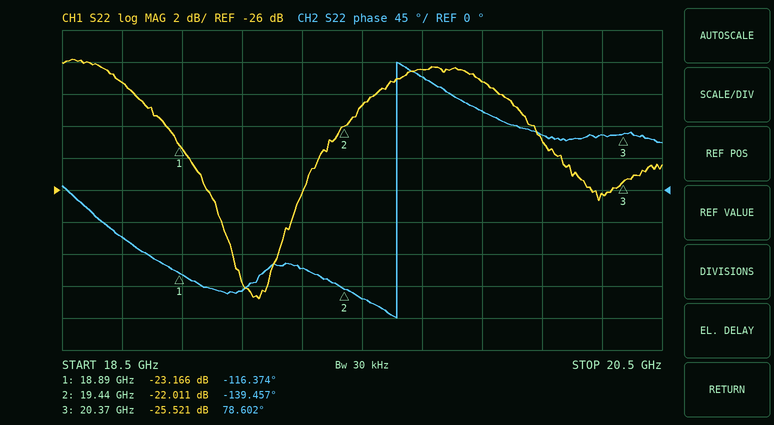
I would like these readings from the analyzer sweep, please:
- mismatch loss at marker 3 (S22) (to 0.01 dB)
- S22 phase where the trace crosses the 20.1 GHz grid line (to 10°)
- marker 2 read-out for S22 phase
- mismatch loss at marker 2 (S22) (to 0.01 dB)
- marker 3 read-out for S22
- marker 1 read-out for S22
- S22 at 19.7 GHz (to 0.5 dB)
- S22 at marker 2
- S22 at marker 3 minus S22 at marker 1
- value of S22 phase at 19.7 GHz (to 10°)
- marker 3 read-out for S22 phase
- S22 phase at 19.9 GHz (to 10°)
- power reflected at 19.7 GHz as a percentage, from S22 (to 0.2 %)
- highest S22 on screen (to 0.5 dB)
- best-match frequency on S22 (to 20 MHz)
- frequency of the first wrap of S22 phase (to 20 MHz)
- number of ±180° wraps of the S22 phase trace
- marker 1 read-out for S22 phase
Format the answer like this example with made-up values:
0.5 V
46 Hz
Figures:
0.01 dB
80°
-139.457°
0.03 dB
-25.521 dB
-23.166 dB
-18.5 dB
-22.011 dB
-2.355 dB
160°
78.602°
110°
1.4 %
-18.0 dB
19.16 GHz
19.62 GHz
1
-116.374°
